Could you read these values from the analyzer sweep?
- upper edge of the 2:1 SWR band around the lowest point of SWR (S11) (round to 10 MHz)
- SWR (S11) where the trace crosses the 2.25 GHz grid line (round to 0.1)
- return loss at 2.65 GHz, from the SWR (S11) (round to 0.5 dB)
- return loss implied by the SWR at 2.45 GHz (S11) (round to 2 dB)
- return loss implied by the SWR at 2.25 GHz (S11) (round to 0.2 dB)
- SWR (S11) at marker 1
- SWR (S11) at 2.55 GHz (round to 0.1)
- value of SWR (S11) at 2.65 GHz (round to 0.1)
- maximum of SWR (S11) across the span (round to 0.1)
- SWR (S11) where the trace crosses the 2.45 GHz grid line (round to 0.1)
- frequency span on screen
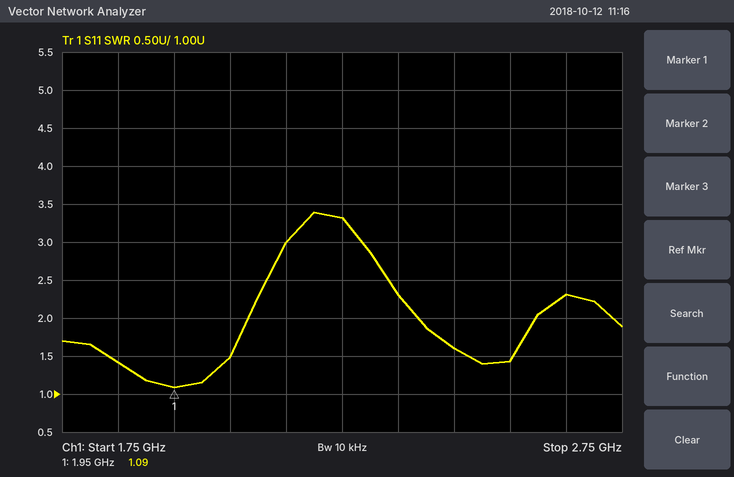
2.08 GHz
3.3
8.0 dB
12 dB
5.4 dB
1.09
1.4
2.3
3.4
1.6
1 GHz
